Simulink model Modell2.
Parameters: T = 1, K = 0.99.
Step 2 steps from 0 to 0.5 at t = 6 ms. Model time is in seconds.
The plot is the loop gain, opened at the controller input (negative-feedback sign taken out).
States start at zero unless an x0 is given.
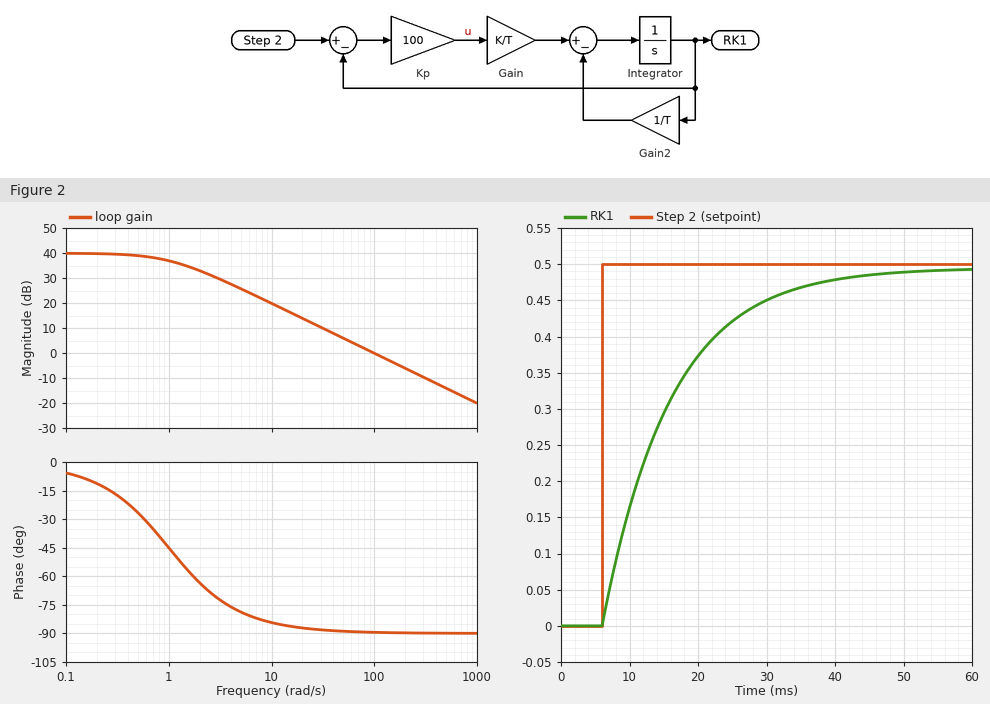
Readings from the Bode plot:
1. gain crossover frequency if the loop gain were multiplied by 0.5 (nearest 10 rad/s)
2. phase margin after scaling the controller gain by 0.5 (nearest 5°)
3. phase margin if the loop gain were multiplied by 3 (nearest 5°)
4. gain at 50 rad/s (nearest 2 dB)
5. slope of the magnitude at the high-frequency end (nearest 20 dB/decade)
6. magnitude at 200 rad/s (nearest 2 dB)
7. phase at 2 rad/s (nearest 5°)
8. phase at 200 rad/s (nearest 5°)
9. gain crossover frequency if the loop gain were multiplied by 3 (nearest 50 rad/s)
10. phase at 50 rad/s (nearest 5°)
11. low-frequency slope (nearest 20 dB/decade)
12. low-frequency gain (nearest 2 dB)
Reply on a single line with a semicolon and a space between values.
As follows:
50 rad/s; 90°; 90°; 6 dB; -20 dB/decade; -6 dB; -65°; -90°; 300 rad/s; -90°; 0 dB/decade; 40 dB
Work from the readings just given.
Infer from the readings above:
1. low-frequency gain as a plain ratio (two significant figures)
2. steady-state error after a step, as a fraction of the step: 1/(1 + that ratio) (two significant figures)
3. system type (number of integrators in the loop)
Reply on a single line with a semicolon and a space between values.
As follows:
100; 0.0099; 0
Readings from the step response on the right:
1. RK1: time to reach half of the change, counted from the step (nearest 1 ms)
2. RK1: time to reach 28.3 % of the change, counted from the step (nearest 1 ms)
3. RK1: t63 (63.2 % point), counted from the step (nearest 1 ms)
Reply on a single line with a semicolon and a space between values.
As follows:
7 ms; 3 ms; 10 ms
